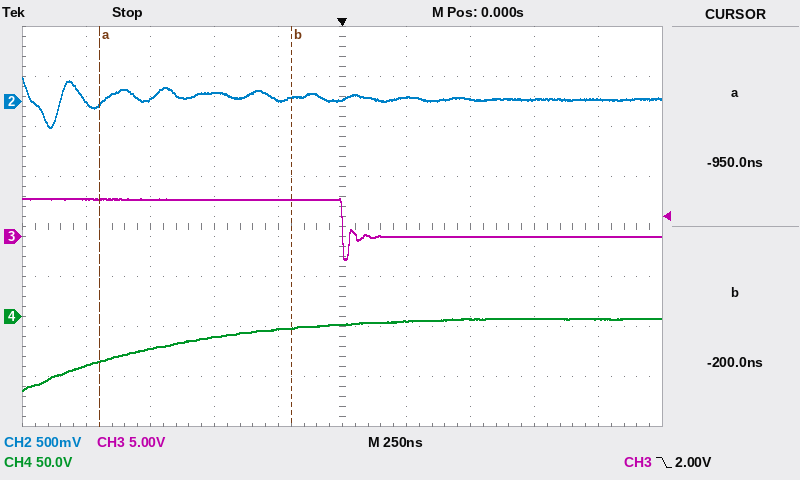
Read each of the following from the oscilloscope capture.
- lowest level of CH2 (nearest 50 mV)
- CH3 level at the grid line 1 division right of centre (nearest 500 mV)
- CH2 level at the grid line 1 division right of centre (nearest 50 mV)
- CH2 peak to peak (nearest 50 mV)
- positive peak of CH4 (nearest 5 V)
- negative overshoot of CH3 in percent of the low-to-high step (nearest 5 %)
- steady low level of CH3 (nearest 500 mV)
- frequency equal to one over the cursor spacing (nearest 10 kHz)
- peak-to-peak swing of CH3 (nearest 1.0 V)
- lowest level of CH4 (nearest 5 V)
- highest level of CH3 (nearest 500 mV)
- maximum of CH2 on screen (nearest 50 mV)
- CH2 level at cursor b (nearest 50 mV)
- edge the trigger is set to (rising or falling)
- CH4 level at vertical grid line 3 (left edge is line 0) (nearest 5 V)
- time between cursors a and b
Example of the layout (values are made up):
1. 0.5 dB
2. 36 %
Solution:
1. -250 mV
2. 0.0 V
3. 50 mV
4. 500 mV
5. 0 V
6. 60 %
7. 0.0 V
8. 1.33 MHz
9. 6.0 V
10. -75 V
11. 4.0 V
12. 250 mV
13. 50 mV
14. falling
15. -20 V
16. 750 ns
